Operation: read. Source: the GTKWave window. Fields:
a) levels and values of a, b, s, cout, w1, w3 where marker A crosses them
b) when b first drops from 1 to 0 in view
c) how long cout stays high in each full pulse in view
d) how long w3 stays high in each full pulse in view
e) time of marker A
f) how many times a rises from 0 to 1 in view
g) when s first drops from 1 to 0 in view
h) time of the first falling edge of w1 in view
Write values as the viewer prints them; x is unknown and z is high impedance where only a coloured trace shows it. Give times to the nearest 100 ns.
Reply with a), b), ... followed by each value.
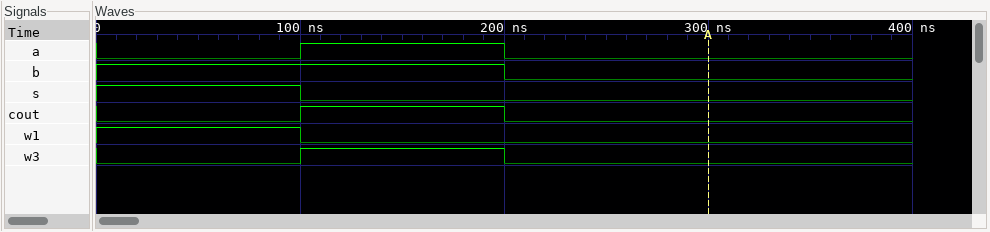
a) a=0, b=0, s=0, cout=0, w1=0, w3=0
b) 200 ns
c) 100 ns
d) 100 ns
e) 300 ns
f) 1
g) 100 ns
h) 100 ns
